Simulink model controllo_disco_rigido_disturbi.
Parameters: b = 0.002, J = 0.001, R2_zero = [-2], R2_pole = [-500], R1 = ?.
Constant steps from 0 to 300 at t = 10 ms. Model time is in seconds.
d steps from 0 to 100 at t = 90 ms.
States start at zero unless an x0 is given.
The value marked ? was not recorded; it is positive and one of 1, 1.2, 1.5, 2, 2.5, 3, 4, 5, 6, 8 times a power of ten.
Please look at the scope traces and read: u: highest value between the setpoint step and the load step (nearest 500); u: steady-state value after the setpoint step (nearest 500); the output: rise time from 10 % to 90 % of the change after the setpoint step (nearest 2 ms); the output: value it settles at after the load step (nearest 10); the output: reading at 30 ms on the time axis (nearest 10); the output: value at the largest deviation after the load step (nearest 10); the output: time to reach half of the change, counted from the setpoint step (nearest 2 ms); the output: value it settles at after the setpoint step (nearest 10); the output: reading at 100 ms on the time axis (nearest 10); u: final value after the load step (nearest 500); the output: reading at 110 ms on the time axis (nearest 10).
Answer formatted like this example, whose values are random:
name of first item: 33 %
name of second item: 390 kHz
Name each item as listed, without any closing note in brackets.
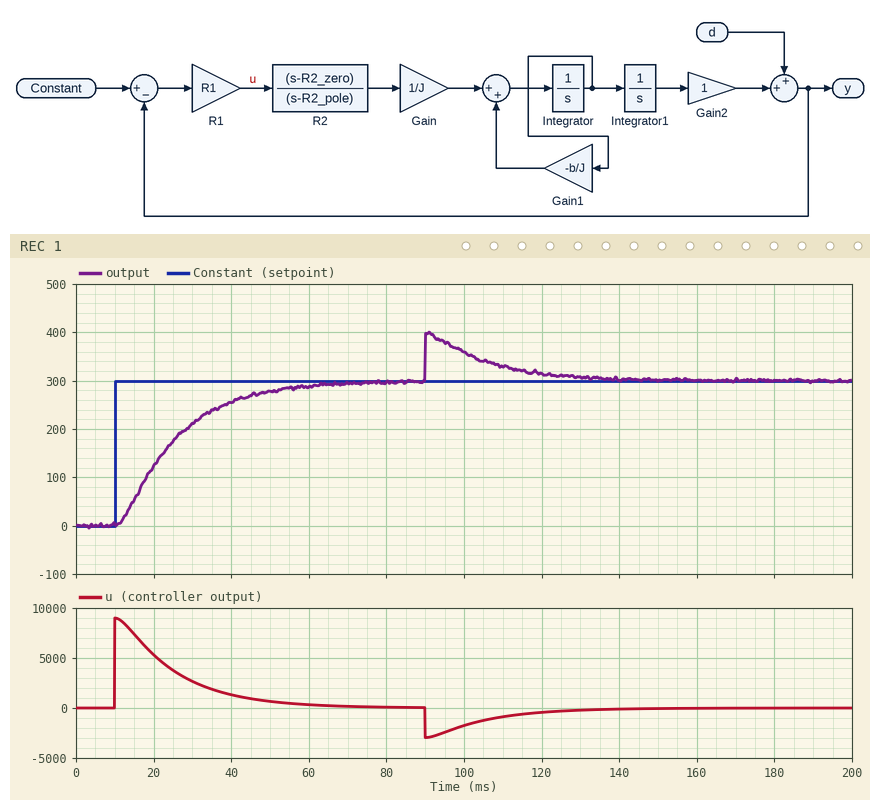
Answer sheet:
u: highest value between the setpoint step and the load step: 9000
u: steady-state value after the setpoint step: 0
the output: rise time from 10 % to 90 % of the change after the setpoint step: 32 ms
the output: value it settles at after the load step: 300
the output: reading at 30 ms on the time axis: 210
the output: value at the largest deviation after the load step: 400
the output: time to reach half of the change, counted from the setpoint step: 12 ms
the output: value it settles at after the setpoint step: 300
the output: reading at 100 ms on the time axis: 360
u: final value after the load step: 0
the output: reading at 110 ms on the time axis: 330
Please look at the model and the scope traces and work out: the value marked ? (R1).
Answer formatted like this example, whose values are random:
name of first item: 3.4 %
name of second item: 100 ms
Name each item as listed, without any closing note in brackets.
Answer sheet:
the value marked ?: 30
